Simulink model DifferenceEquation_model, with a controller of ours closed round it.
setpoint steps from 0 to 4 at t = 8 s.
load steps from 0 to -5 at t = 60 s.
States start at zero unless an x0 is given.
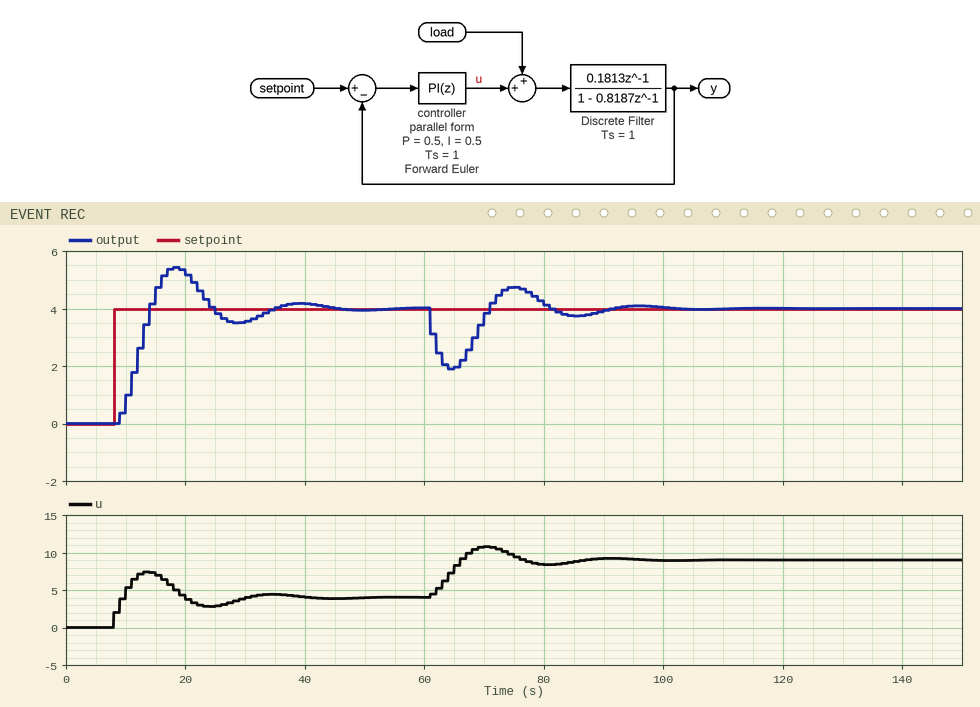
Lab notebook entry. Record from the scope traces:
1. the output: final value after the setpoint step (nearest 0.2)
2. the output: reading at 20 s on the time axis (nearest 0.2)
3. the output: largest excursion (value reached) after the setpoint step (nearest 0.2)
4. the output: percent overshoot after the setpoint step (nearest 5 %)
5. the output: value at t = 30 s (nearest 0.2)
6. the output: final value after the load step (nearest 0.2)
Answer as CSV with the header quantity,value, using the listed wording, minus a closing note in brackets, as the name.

quantity,value
the output: final value after the setpoint step,4.0
the output: reading at 20 s on the time axis,5.2
the output: largest excursion (value reached) after the setpoint step,5.4
the output: percent overshoot after the setpoint step,35 %
the output: value at t = 30 s,3.6
the output: final value after the load step,4.0
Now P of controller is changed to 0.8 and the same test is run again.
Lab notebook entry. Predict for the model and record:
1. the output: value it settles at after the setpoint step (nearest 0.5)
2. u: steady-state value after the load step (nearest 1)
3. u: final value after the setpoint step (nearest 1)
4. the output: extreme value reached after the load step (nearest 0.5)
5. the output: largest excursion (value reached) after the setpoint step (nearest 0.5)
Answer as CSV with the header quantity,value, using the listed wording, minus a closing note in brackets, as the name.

quantity,value
the output: value it settles at after the setpoint step,4.0
u: steady-state value after the load step,9
u: final value after the setpoint step,4
the output: extreme value reached after the load step,2.0
the output: largest excursion (value reached) after the setpoint step,5.0
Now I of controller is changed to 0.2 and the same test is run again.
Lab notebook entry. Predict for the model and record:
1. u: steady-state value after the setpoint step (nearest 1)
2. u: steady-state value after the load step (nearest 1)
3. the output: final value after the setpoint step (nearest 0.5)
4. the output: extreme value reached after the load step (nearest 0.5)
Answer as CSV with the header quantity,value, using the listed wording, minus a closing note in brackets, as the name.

quantity,value
u: steady-state value after the setpoint step,4
u: steady-state value after the load step,9
the output: final value after the setpoint step,4.0
the output: extreme value reached after the load step,1.5
